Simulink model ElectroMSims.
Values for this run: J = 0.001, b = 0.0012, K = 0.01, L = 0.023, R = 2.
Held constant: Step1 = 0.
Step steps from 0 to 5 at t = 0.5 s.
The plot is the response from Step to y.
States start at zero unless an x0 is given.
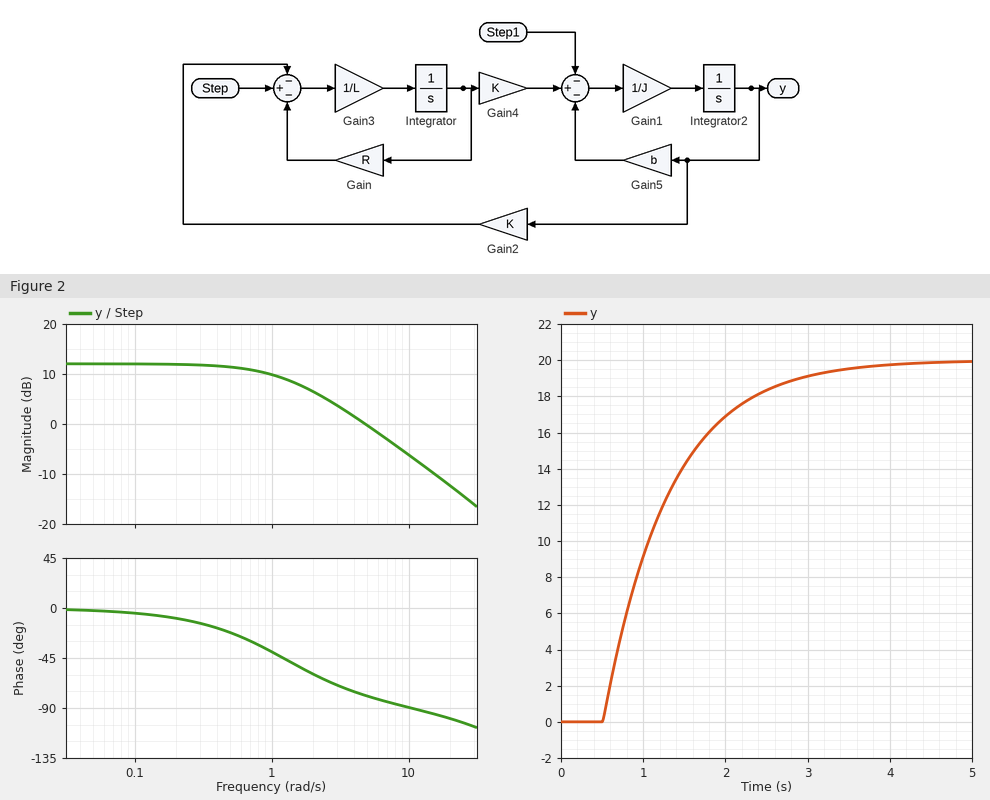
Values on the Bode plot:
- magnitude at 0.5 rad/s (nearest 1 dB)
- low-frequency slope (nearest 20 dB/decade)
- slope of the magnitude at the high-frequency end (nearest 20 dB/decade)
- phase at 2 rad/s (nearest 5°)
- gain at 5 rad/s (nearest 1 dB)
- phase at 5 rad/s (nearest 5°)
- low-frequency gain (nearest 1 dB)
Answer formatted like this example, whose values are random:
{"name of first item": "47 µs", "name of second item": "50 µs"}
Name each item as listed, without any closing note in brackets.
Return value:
{"magnitude at 0.5 rad/s": "11 dB", "low-frequency slope": "0 dB/decade", "slope of the magnitude at the high-frequency end": "-20 dB/decade", "phase at 2 rad/s": "-60°", "gain at 5 rad/s": "0 dB", "phase at 5 rad/s": "-80°", "low-frequency gain": "12 dB"}
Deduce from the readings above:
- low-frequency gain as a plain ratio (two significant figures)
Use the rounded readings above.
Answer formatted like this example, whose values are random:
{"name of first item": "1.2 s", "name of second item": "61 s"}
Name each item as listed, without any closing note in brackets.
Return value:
{"low-frequency gain as a plain ratio": "4.0"}
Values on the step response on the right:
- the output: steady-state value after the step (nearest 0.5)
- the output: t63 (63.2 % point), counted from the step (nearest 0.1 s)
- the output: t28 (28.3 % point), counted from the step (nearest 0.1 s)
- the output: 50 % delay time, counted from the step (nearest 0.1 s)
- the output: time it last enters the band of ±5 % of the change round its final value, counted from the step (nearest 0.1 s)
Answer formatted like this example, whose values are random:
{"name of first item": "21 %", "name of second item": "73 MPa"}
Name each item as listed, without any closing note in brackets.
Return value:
{"the output: steady-state value after the step": "20.0", "the output: t63 (63.2 % point), counted from the step": "0.8 s", "the output: t28 (28.3 % point), counted from the step": "0.3 s", "the output: 50 % delay time, counted from the step": "0.6 s", "the output: time it last enters the band of ±5 % of the change round its final value, counted from the step": "2.4 s"}
